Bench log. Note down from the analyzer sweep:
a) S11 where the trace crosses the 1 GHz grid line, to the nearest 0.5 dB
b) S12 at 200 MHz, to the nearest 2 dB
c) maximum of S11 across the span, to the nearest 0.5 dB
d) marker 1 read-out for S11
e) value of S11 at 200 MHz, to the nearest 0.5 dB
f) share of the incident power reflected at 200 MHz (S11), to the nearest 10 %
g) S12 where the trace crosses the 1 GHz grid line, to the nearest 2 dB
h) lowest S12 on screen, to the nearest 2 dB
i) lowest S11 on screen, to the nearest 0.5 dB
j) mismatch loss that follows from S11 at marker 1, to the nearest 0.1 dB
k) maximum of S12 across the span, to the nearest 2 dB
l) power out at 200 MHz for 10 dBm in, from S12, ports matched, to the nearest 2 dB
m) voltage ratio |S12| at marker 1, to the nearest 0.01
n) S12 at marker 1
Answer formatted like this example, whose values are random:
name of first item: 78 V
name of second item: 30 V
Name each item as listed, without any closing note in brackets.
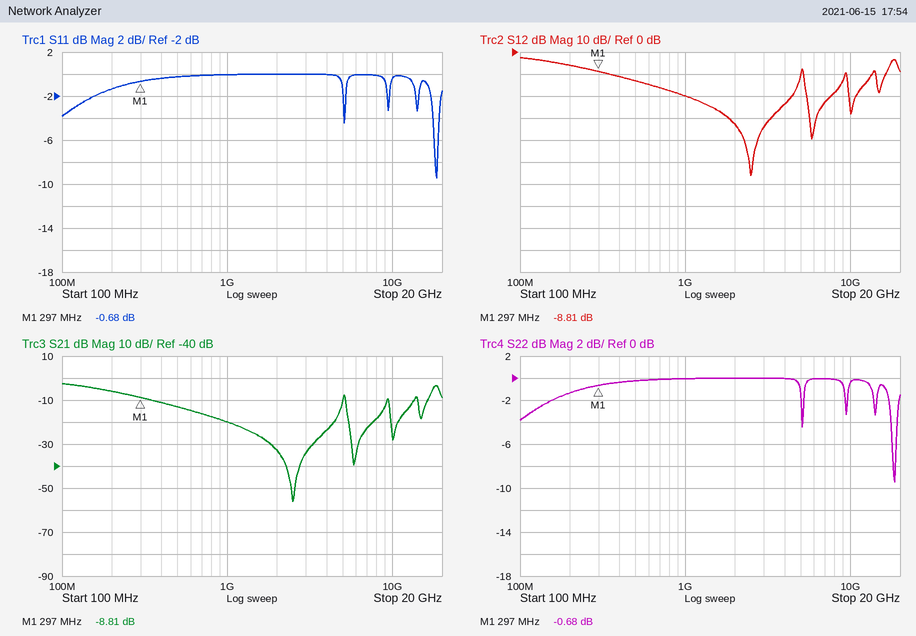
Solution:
S11 where the trace crosses the 1 GHz grid line, to the nearest 0.5 dB: 0.0 dB
S12 at 200 MHz, to the nearest 2 dB: -6 dB
maximum of S11 across the span, to the nearest 0.5 dB: 0.0 dB
marker 1 read-out for S11: -0.68 dB
value of S11 at 200 MHz, to the nearest 0.5 dB: -1.5 dB
share of the incident power reflected at 200 MHz (S11), to the nearest 10 %: 70 %
S12 where the trace crosses the 1 GHz grid line, to the nearest 2 dB: -20 dB
lowest S12 on screen, to the nearest 2 dB: -56 dB
lowest S11 on screen, to the nearest 0.5 dB: -9.5 dB
mismatch loss that follows from S11 at marker 1, to the nearest 0.1 dB: 8.4 dB
maximum of S12 across the span, to the nearest 2 dB: -2 dB
power out at 200 MHz for 10 dBm in, from S12, ports matched, to the nearest 2 dB: 4 dBm
voltage ratio |S12| at marker 1, to the nearest 0.01: 0.36
S12 at marker 1: -8.81 dB
